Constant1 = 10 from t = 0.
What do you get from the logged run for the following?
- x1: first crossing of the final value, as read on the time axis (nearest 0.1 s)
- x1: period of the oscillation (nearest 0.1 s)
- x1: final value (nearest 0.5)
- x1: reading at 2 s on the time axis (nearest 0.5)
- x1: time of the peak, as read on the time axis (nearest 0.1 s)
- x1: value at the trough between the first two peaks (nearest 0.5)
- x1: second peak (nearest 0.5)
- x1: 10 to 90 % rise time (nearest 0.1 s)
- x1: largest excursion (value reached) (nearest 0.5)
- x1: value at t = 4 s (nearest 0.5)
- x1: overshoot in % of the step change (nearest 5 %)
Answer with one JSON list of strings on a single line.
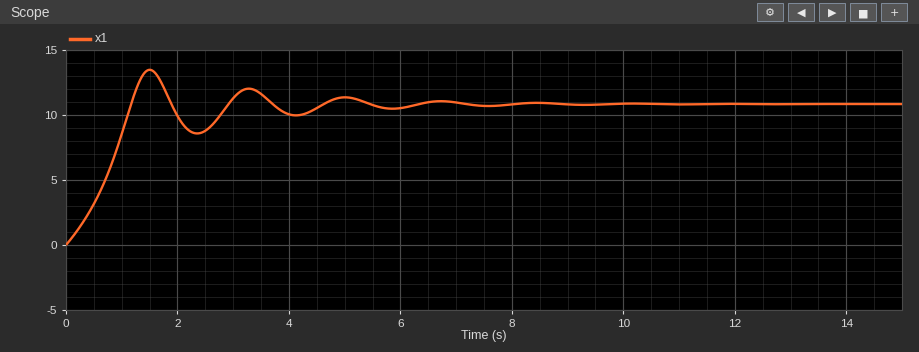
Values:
["1.2 s", "1.8 s", "11.0", "10.0", "1.5 s", "8.5", "12.0", "0.9 s", "13.5", "10.0", "25 %"]
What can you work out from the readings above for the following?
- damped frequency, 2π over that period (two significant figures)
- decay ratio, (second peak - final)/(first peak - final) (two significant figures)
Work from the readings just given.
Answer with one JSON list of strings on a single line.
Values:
["3.5 rad/s", "0.40"]
